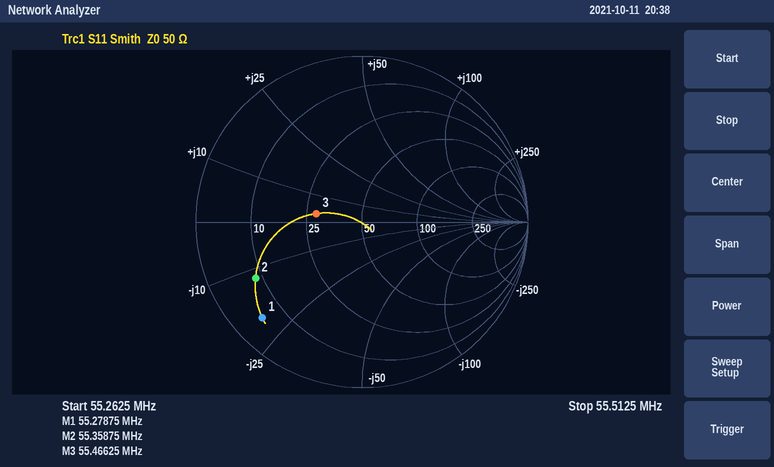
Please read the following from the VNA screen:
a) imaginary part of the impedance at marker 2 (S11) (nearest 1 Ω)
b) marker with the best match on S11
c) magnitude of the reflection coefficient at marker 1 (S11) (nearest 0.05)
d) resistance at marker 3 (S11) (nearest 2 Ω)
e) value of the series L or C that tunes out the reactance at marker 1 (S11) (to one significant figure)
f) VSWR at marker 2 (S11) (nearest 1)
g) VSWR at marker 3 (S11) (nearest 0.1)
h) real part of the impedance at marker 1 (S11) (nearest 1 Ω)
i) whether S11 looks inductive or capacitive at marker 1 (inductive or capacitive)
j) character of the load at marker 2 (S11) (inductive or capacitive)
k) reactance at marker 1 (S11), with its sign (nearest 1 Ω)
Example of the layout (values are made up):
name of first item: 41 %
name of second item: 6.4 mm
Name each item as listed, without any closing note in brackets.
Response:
imaginary part of the impedance at marker 2 (S11): -12 Ω
marker with the best match on S11: marker 3
magnitude of the reflection coefficient at marker 1 (S11): 0.85
resistance at marker 3 (S11): 28 Ω
value of the series L or C that tunes out the reactance at marker 1 (S11): 60 nH
VSWR at marker 2 (S11): 6
VSWR at marker 3 (S11): 1.8
real part of the impedance at marker 1 (S11): 5 Ω
whether S11 looks inductive or capacitive at marker 1: capacitive
character of the load at marker 2 (S11): capacitive
reactance at marker 1 (S11), with its sign: -20 Ω
